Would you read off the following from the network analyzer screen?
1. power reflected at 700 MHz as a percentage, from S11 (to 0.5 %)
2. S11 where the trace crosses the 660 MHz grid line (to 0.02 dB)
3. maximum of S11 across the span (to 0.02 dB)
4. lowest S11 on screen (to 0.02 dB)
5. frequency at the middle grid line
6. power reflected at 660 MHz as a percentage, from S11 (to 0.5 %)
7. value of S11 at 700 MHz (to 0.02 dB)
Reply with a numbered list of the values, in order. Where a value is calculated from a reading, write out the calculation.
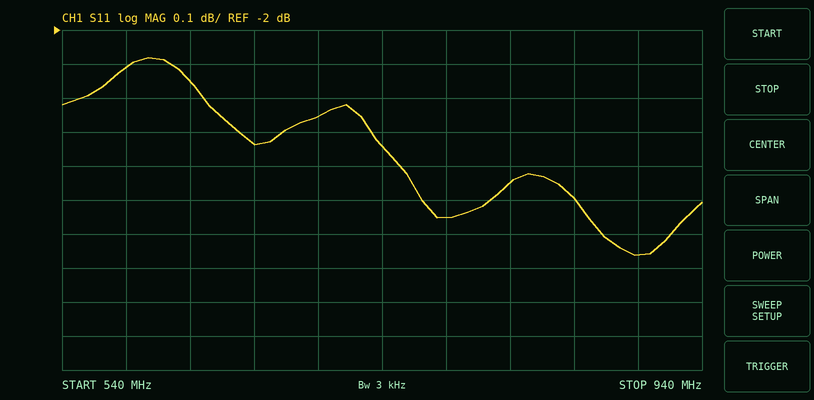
1. 10^(-2.26/10) ≈ 59.4 %, so 59.5 % to the nearest 0.5 %
2. -2.34 dB
3. -2.08 dB
4. -2.66 dB
5. 740 MHz
6. 10^(-2.34/10) ≈ 58.3 %, so 58.5 % to the nearest 0.5 %
7. -2.26 dB
